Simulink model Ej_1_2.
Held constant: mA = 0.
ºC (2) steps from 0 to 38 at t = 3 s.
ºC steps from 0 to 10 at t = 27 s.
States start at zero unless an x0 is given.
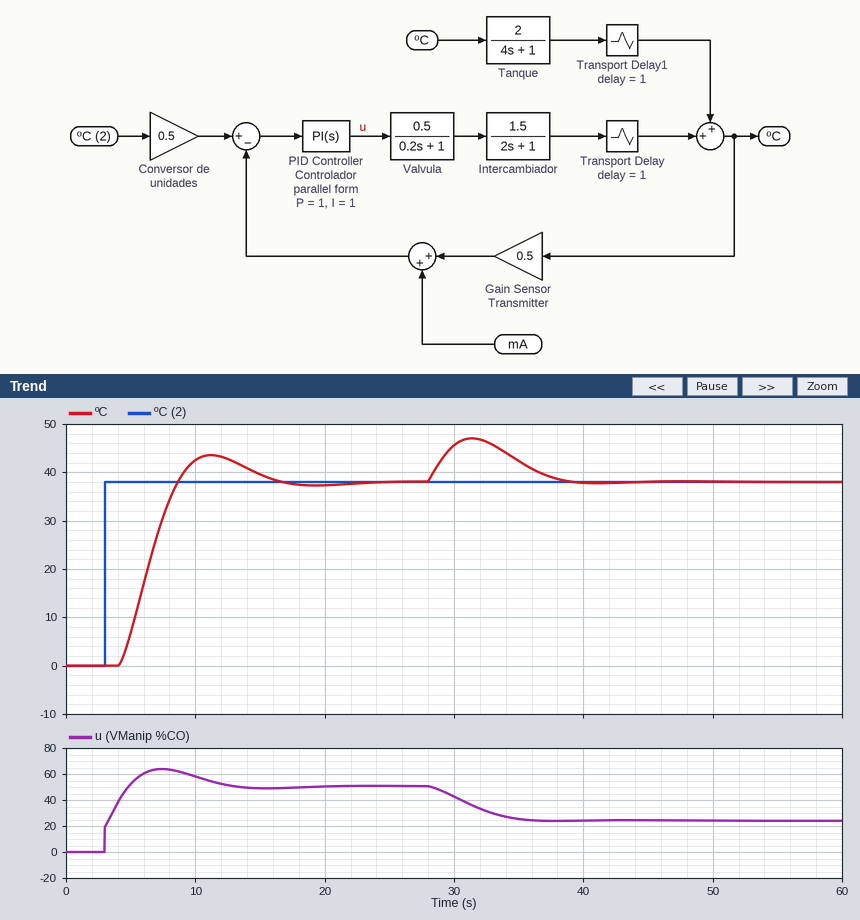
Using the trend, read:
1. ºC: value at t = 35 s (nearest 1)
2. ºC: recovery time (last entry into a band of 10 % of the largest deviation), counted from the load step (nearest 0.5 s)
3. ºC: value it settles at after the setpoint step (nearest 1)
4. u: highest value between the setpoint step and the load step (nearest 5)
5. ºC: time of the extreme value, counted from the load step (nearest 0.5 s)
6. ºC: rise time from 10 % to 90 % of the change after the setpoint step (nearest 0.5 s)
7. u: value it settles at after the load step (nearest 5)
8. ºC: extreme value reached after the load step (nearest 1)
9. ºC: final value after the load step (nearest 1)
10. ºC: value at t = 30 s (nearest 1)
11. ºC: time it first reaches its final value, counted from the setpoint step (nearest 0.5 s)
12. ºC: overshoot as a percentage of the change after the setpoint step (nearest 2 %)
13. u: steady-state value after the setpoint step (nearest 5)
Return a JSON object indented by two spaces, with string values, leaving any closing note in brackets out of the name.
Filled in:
{
  "ºC: value at t = 35 s": "42",
  "ºC: recovery time (last entry into a band of 10 % of the largest deviation), counted from the load step": "10.5 s",
  "ºC: value it settles at after the setpoint step": "38",
  "u: highest value between the setpoint step and the load step": "65",
  "ºC: time of the extreme value, counted from the load step": "4.5 s",
  "ºC: rise time from 10 % to 90 % of the change after the setpoint step": "3.5 s",
  "u: value it settles at after the load step": "25",
  "ºC: extreme value reached after the load step": "47",
  "ºC: final value after the load step": "38",
  "ºC: value at t = 30 s": "46",
  "ºC: time it first reaches its final value, counted from the setpoint step": "5.5 s",
  "ºC: overshoot as a percentage of the change after the setpoint step": "14 %",
  "u: steady-state value after the setpoint step": "50"
}
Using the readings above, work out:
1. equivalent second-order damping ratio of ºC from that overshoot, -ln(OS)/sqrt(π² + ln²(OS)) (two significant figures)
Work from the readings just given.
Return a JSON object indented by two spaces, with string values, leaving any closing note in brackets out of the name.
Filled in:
{
  "equivalent second-order damping ratio of ºC from that overshoot, -ln(OS)/sqrt(π² + ln²(OS))": "0.53"
}
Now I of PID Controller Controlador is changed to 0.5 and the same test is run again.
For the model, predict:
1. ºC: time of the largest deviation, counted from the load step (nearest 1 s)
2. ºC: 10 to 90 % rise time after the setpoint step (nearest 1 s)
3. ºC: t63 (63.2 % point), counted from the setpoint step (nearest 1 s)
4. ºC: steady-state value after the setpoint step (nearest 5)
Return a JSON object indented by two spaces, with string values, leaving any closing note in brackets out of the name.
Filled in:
{
  "ºC: time of the largest deviation, counted from the load step": "5 s",
  "ºC: 10 to 90 % rise time after the setpoint step": "9 s",
  "ºC: t63 (63.2 % point), counted from the setpoint step": "5 s",
  "ºC: steady-state value after the setpoint step": "40"
}
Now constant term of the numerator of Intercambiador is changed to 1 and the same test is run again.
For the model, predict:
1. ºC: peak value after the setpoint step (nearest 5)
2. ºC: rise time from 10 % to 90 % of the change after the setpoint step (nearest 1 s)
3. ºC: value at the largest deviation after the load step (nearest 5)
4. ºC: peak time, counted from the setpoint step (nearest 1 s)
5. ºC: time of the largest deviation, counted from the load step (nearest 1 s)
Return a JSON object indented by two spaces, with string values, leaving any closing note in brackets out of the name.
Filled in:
{
  "ºC: peak value after the setpoint step": "40",
  "ºC: rise time from 10 % to 90 % of the change after the setpoint step": "5 s",
  "ºC: value at the largest deviation after the load step": "50",
  "ºC: peak time, counted from the setpoint step": "12 s",
  "ºC: time of the largest deviation, counted from the load step": "5 s"
}
